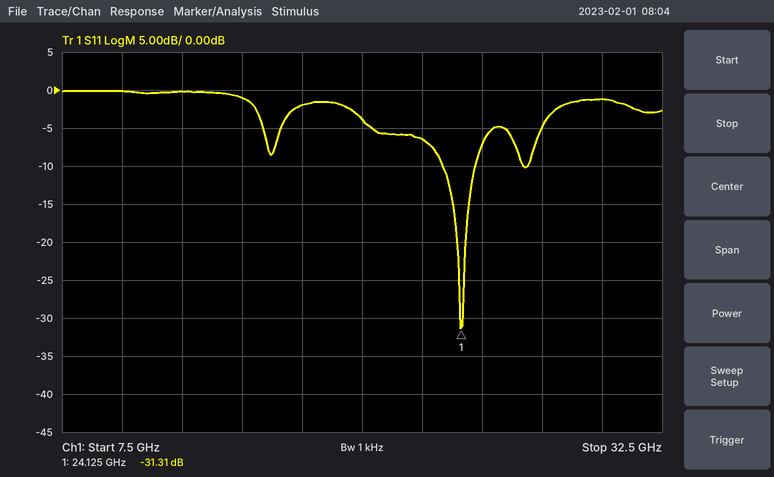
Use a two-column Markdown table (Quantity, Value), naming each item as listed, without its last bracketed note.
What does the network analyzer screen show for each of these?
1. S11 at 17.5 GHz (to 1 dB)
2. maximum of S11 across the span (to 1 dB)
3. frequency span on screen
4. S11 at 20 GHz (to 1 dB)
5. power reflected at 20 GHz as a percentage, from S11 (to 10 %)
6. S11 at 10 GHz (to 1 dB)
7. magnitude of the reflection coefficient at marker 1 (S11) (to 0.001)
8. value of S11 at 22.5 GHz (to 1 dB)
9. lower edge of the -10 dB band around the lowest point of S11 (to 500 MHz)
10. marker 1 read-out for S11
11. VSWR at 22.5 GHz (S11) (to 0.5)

| Quantity | Value |
|---|---|
| S11 at 17.5 GHz | -2 dB |
| maximum of S11 across the span | 0 dB |
| frequency span on screen | 25 GHz |
| S11 at 20 GHz | -4 dB |
| power reflected at 20 GHz as a percentage, from S11 | 40 % |
| S11 at 10 GHz | 0 dB |
| magnitude of the reflection coefficient at marker 1 (S11) | 0.027 |
| value of S11 at 22.5 GHz | -6 dB |
| lower edge of the -10 dB band around the lowest point of S11 | 23.5 GHz |
| marker 1 read-out for S11 | -31.31 dB |
| VSWR at 22.5 GHz (S11) | 3.0 |
